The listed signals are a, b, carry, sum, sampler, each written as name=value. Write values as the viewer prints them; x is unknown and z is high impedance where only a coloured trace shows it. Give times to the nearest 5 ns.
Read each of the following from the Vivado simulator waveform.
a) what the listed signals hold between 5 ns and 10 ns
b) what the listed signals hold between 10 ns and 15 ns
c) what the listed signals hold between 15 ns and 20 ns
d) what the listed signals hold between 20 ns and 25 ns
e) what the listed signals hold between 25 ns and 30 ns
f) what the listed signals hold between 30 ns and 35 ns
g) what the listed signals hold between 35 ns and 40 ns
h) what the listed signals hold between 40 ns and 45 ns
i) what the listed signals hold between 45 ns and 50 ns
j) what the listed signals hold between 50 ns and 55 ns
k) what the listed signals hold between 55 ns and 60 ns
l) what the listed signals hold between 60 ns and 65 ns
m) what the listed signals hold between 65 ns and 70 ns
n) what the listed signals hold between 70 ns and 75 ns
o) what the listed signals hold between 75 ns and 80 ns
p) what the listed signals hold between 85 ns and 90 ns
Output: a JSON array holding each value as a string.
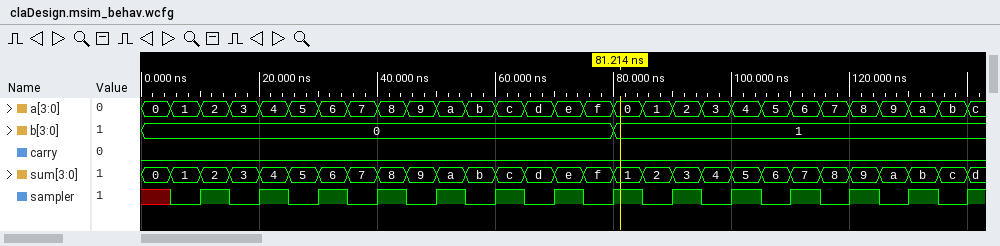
["a=1, b=0, carry=0, sum=1, sampler=0", "a=2, b=0, carry=0, sum=2, sampler=1", "a=3, b=0, carry=0, sum=3, sampler=0", "a=4, b=0, carry=0, sum=4, sampler=1", "a=5, b=0, carry=0, sum=5, sampler=0", "a=6, b=0, carry=0, sum=6, sampler=1", "a=7, b=0, carry=0, sum=7, sampler=0", "a=8, b=0, carry=0, sum=8, sampler=1", "a=9, b=0, carry=0, sum=9, sampler=0", "a=a, b=0, carry=0, sum=a, sampler=1", "a=b, b=0, carry=0, sum=b, sampler=0", "a=c, b=0, carry=0, sum=c, sampler=1", "a=d, b=0, carry=0, sum=d, sampler=0", "a=e, b=0, carry=0, sum=e, sampler=1", "a=f, b=0, carry=0, sum=f, sampler=0", "a=1, b=1, carry=0, sum=2, sampler=0"]
